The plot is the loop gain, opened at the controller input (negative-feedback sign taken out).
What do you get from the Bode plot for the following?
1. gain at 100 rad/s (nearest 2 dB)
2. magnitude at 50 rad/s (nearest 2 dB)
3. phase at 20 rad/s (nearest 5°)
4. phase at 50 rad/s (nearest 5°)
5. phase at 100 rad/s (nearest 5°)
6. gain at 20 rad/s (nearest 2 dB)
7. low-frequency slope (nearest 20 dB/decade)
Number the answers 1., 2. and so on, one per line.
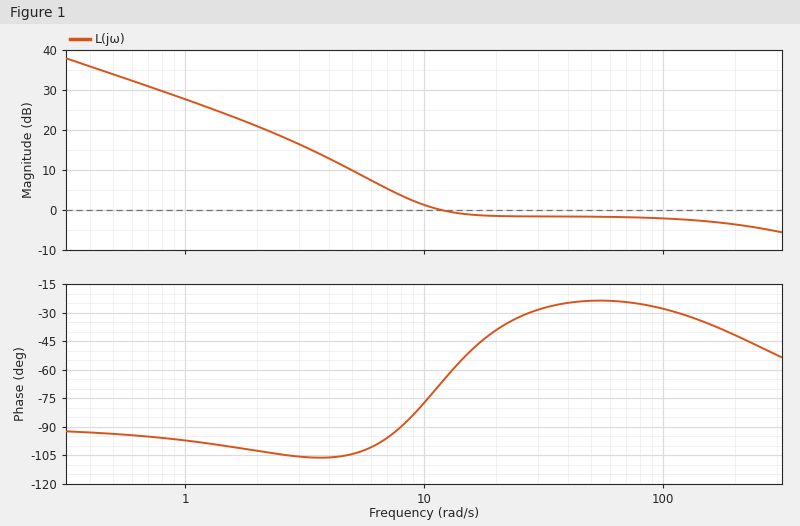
1. -2 dB
2. -2 dB
3. -40°
4. -25°
5. -30°
6. -2 dB
7. -20 dB/decade
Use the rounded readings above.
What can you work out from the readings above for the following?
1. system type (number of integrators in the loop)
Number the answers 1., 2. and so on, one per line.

1. 1
